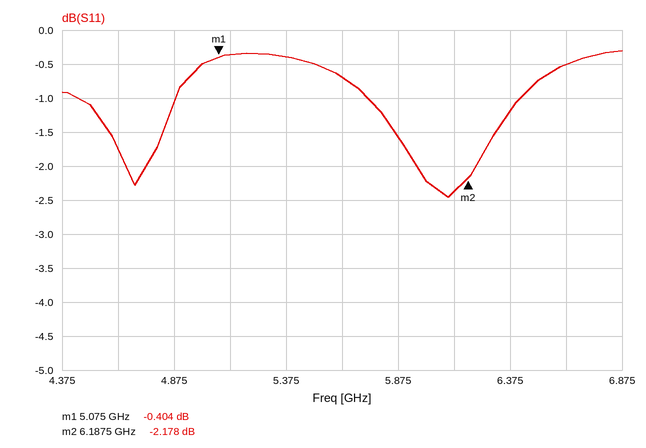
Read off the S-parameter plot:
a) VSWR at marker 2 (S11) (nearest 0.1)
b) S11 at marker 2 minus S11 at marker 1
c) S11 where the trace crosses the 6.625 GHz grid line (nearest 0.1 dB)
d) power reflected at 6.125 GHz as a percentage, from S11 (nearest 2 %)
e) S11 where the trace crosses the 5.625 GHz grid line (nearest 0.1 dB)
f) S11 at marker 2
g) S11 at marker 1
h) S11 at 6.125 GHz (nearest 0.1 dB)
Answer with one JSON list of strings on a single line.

["8.0", "-1.774 dB", "-0.5 dB", "58 %", "-0.7 dB", "-2.178 dB", "-0.404 dB", "-2.4 dB"]
